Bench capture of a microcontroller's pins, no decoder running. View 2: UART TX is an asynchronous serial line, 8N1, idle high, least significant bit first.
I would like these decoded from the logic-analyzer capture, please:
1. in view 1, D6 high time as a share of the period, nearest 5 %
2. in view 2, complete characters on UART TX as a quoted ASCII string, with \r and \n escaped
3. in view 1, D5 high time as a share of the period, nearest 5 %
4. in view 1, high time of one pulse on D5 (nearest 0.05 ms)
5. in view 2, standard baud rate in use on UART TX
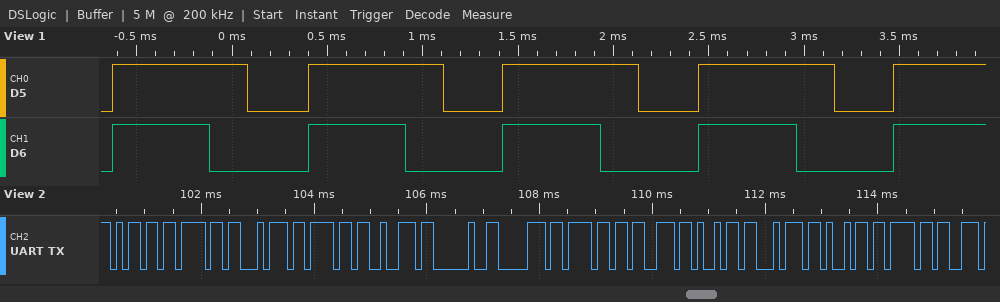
50 %
"motor positio"
70 %
0.70 ms
9600 baud
